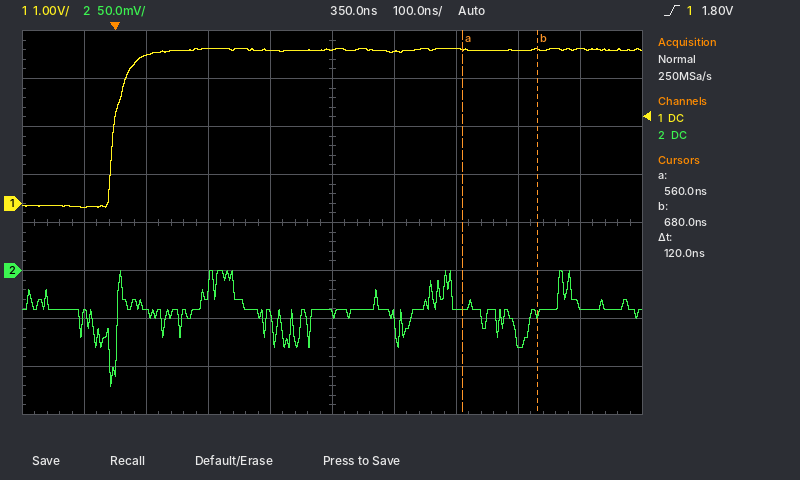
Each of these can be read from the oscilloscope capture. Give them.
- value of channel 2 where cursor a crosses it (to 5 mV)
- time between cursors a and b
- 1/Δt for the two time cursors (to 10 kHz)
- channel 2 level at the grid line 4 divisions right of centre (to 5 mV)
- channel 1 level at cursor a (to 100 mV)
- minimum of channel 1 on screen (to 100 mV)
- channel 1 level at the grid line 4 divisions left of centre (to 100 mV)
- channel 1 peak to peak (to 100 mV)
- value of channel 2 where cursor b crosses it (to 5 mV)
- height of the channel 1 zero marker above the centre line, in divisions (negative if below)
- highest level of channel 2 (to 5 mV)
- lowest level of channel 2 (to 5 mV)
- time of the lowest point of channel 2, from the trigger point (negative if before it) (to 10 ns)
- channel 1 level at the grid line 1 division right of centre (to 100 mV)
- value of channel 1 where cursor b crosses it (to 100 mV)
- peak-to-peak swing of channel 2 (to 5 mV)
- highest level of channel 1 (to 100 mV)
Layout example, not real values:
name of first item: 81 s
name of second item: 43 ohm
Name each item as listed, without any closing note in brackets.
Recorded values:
value of channel 2 where cursor a crosses it: -40 mV
time between cursors a and b: 120 ns
1/Δt for the two time cursors: 8.33 MHz
channel 2 level at the grid line 4 divisions right of centre: -35 mV
channel 1 level at cursor a: 3.2 V
minimum of channel 1 on screen: -100 mV
channel 1 level at the grid line 4 divisions left of centre: -100 mV
channel 1 peak to peak: 3.3 V
value of channel 2 where cursor b crosses it: -45 mV
height of the channel 1 zero marker above the centre line, in divisions: +0.4 div
highest level of channel 2: 0 mV
lowest level of channel 2: -120 mV
time of the lowest point of channel 2, from the trigger point (negative if before it): -10 ns
channel 1 level at the grid line 1 division right of centre: 3.2 V
value of channel 1 where cursor b crosses it: 3.2 V
peak-to-peak swing of channel 2: 120 mV
highest level of channel 1: 3.2 V
